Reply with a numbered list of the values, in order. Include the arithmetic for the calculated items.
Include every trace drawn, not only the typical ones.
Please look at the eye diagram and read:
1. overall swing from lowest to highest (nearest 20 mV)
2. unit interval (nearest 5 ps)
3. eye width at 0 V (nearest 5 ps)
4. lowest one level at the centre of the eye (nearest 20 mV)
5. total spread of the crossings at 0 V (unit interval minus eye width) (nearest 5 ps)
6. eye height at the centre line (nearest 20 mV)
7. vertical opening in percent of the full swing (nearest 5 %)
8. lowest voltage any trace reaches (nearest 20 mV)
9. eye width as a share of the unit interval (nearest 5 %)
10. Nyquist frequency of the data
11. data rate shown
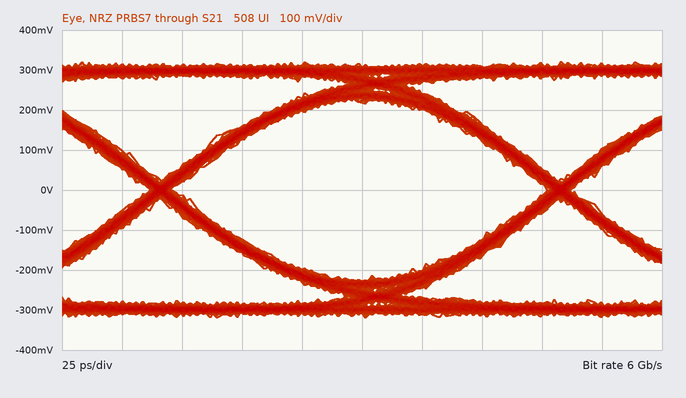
1. 640 mV
2. 165 ps
3. 155 ps
4. 220 mV
5. 10 ps
6. 440 mV
7. 440 mV / 640 mV ≈ 68.8 %, so 70 % to the nearest 5 %
8. -320 mV
9. 155 ps / 165 ps ≈ 93.9 %, so 95 % to the nearest 5 %
10. 3 GHz
11. 6 Gb/s
